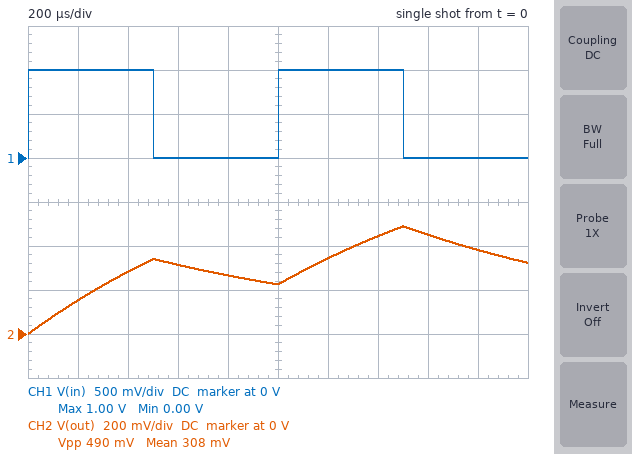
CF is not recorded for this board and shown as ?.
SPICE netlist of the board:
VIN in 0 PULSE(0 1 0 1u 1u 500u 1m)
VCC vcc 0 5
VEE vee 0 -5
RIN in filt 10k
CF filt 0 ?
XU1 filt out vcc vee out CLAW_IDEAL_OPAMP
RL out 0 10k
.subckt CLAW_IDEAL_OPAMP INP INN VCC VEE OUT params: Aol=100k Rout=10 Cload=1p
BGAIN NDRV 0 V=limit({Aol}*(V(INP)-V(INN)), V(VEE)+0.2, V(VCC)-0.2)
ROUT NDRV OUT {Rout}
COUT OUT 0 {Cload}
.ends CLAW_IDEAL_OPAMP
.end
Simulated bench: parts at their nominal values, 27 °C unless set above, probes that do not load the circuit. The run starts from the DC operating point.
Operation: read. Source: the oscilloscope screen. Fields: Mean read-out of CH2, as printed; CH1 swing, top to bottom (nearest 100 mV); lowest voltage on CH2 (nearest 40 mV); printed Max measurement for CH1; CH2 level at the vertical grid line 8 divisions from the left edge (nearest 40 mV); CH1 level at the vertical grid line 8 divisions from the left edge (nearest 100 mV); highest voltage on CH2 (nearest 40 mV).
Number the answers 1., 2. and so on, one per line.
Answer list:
1. 308 mV
2. 1.0 V
3. 0 V
4. 1.00 V
5. 440 mV
6. 0 V
7. 480 mV
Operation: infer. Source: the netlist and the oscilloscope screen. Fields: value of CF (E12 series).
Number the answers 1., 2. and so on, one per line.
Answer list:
1. 120 nF
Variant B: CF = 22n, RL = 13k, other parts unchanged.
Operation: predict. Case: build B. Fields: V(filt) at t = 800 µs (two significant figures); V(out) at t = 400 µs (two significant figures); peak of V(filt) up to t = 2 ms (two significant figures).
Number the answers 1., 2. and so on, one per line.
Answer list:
1. 230 mV
2. 840 mV
3. 910 mV
